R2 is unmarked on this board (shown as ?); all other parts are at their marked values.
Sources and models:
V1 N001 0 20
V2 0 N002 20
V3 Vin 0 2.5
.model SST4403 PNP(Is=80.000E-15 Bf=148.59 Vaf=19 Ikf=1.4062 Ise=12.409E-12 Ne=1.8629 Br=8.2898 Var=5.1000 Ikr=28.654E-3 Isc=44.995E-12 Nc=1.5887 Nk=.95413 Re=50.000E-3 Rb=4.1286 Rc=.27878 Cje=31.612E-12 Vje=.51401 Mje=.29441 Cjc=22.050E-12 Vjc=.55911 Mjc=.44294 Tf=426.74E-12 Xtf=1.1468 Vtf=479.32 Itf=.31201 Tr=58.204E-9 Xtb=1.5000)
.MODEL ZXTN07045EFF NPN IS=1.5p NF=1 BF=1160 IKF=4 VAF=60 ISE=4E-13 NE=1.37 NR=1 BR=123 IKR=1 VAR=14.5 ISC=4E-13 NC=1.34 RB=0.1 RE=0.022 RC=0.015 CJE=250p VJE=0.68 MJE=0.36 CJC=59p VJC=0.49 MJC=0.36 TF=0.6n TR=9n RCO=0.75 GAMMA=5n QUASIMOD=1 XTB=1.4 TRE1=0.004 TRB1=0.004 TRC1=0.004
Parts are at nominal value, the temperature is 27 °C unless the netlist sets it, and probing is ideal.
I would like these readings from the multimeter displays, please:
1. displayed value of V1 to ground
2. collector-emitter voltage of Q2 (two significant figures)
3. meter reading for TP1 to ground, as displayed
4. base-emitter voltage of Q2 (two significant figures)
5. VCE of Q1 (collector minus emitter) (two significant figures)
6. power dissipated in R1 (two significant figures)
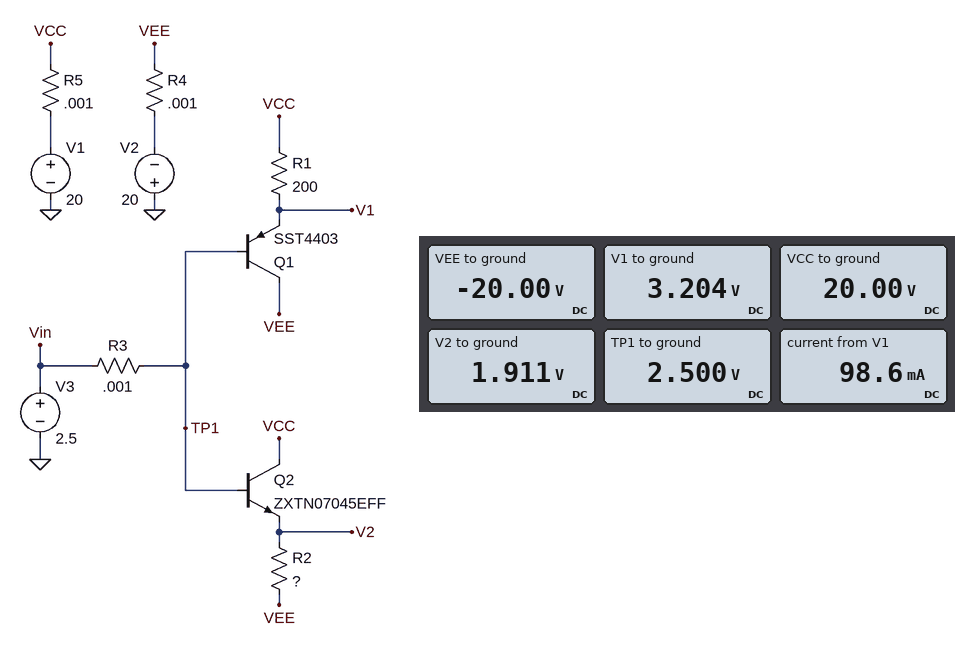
3.204 V
18 V
2.500 V
590 mV
-23 V
1.4 W
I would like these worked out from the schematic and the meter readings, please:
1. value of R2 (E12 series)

1.5 kΩ
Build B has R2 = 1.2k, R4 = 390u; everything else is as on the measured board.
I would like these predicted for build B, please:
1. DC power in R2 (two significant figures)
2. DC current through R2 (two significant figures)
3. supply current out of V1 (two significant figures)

400 mW
18 mA
100 mA
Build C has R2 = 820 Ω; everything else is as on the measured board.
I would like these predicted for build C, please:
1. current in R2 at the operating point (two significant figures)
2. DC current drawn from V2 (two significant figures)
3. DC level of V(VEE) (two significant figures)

27 mA
110 mA
-20 V
